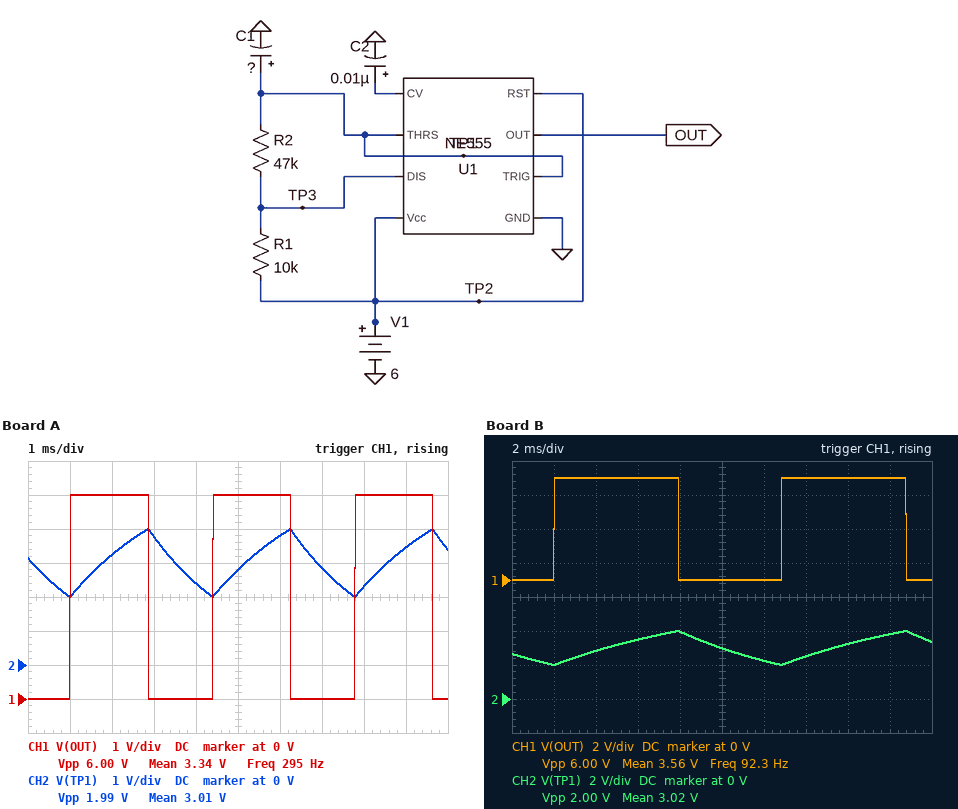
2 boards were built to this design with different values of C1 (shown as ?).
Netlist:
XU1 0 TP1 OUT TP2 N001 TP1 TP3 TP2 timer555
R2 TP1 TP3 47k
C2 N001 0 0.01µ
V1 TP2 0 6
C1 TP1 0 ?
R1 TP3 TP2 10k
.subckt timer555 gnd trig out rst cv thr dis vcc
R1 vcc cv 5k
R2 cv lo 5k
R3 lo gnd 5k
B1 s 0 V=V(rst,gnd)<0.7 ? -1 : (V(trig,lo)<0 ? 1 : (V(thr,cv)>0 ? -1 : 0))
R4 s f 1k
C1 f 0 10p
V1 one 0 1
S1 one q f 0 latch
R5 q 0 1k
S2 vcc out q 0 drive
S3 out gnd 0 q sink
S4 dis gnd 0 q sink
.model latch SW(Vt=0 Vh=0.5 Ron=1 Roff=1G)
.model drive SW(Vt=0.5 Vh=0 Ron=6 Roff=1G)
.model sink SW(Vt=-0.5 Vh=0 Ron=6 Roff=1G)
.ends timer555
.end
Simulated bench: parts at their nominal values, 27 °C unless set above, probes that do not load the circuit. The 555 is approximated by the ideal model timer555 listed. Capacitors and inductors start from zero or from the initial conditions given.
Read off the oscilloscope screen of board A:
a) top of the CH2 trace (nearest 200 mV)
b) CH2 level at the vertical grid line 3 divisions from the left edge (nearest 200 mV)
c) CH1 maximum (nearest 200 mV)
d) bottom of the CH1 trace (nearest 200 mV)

4.0 V
3.8 V
6.0 V
0 V
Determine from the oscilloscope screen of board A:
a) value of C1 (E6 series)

47 nF
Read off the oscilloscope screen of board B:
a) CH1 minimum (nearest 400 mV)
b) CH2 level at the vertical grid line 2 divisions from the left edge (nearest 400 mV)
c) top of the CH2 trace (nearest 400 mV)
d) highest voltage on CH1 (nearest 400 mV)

0 V
2.8 V
4.0 V
6.0 V
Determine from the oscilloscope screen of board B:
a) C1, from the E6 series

150 nF
